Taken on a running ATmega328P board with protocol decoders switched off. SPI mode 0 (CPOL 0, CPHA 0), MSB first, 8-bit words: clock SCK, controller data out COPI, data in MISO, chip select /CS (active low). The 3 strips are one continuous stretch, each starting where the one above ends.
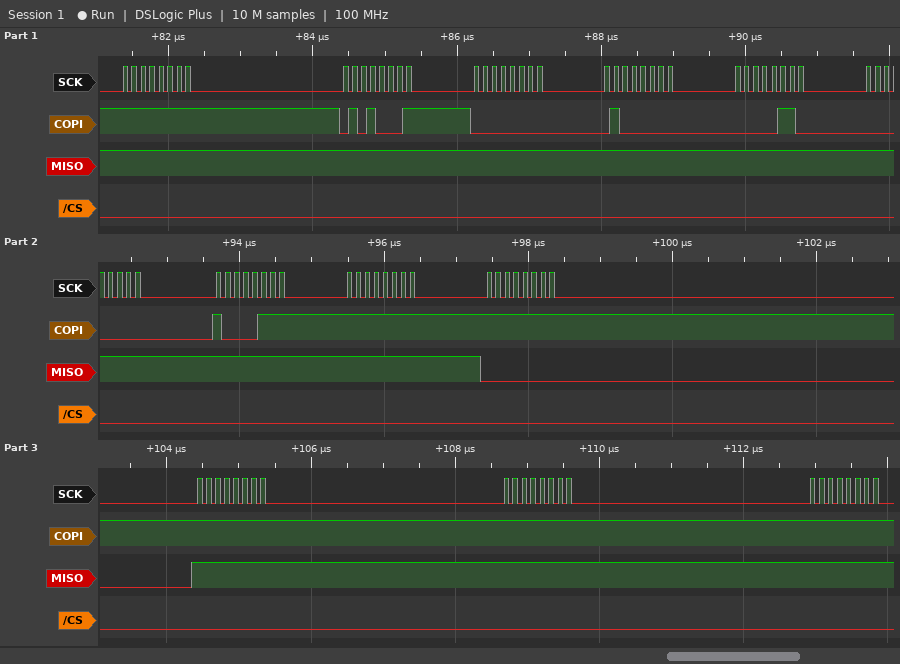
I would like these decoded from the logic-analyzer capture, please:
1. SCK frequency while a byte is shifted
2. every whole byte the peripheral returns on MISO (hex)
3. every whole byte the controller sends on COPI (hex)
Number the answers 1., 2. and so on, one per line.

1. 8 MHz
2. FF FF FF FF FF FF FF FF 00 FF FF FF
3. FF 51 00 40 06 00 87 FF FF FF FF FF
